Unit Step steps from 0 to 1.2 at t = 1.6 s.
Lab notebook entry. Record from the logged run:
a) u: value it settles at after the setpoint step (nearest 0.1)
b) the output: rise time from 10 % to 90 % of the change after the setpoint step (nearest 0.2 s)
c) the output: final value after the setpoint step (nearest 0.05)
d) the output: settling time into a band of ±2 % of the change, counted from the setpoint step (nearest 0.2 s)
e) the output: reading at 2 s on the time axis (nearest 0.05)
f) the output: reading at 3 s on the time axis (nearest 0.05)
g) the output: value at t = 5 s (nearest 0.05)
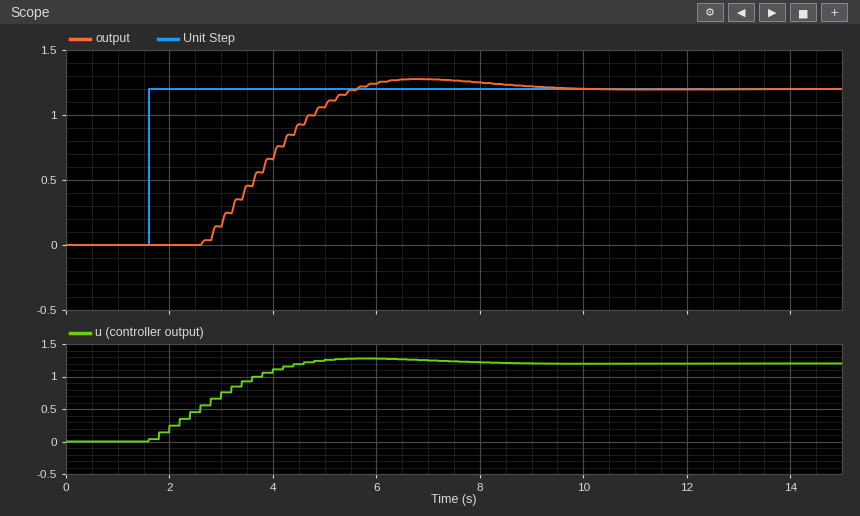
1.2
2.2 s
1.20
7.2 s
0.00
0.15
1.05
